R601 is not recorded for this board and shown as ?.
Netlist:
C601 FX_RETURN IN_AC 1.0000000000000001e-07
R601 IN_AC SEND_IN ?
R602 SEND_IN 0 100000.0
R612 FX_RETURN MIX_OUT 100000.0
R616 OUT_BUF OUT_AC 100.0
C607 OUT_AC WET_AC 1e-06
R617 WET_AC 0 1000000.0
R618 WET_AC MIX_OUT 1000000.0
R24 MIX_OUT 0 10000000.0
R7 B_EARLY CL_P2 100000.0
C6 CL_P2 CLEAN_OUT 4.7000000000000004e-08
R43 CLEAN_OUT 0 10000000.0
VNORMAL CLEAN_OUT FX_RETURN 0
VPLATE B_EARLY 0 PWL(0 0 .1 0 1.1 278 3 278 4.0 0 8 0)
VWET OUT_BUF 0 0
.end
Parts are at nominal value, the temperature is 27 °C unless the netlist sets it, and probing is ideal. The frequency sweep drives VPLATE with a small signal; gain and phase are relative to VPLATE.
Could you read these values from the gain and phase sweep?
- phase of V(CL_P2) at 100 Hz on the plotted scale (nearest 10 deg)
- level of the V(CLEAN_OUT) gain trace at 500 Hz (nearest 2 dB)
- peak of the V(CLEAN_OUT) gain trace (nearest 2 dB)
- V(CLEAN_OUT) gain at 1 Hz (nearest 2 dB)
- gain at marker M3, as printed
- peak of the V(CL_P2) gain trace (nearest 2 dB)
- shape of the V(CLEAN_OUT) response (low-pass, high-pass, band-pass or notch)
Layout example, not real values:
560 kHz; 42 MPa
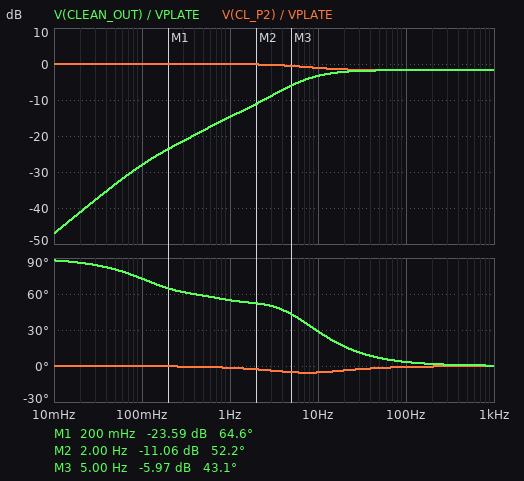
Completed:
0 deg; -2 dB; -2 dB; -14 dB; -5.97 dB; 0 dB; high-pass
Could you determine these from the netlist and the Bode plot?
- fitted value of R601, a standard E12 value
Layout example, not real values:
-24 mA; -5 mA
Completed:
820 kΩ
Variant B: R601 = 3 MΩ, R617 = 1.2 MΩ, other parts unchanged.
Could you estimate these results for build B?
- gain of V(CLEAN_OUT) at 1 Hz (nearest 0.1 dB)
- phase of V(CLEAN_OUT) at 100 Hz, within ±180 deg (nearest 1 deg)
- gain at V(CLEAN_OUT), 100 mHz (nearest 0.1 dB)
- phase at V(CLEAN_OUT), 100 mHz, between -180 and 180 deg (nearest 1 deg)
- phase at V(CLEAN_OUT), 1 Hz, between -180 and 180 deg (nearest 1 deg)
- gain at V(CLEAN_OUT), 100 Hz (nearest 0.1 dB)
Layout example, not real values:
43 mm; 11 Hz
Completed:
-13.7 dB; 2 deg; -27.9 dB; 71 deg; 66 deg; -1.2 dB
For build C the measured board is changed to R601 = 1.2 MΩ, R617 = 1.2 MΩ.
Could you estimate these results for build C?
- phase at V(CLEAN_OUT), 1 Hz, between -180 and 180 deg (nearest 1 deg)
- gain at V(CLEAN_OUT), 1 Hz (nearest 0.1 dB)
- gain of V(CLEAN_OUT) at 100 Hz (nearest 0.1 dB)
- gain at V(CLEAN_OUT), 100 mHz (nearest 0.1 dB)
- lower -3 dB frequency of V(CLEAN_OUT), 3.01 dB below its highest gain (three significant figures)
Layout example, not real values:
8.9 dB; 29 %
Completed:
58 deg; -14.6 dB; -1.5 dB; -27.8 dB; 5.67 Hz
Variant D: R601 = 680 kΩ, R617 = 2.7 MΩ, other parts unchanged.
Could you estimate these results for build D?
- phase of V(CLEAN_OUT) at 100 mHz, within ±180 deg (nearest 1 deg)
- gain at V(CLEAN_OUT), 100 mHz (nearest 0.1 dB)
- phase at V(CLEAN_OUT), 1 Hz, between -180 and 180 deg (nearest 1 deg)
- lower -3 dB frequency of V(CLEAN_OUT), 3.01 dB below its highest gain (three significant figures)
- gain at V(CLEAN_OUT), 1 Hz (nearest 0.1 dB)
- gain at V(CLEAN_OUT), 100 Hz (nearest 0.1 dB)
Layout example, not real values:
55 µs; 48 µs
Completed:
59 deg; -27.2 dB; 53 deg; 7.09 Hz; -14.8 dB; -1.9 dB
